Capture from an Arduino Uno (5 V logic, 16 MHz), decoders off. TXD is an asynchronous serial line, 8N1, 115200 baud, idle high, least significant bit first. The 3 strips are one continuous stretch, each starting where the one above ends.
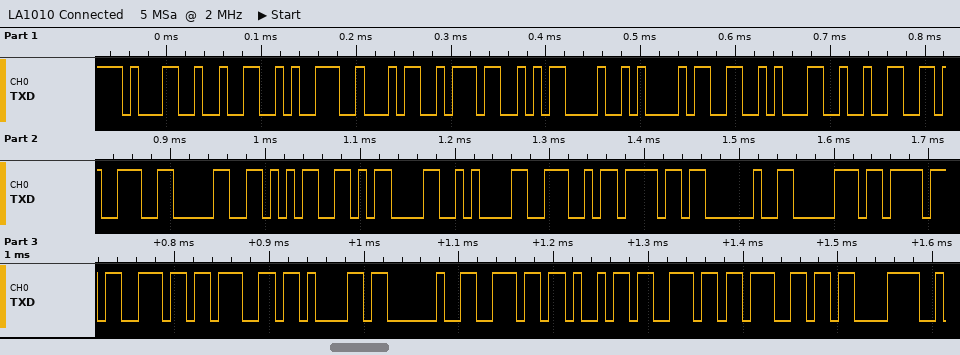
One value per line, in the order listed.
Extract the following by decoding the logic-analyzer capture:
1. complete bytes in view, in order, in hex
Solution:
31 32 39 34 37 0D 0A 33 31 32 39 30 35 0D 0A 4E 6F 20 70 6F 6E 67 61 20 6E 69 6E 67 C3
